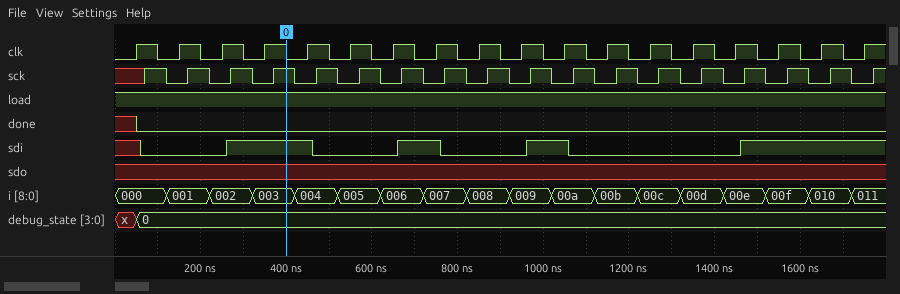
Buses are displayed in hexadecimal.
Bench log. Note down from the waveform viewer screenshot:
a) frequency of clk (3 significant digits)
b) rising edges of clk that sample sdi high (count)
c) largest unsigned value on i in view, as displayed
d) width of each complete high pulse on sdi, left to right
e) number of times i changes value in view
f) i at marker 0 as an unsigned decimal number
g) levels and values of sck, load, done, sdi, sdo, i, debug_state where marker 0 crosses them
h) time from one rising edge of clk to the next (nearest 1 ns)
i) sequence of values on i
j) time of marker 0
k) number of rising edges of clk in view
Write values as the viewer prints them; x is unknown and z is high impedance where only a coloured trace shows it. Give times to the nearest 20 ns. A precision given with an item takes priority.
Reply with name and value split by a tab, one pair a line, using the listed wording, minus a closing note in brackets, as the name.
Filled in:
frequency of clk	10.0 MHz
rising edges of clk that sample sdi high	7
largest unsigned value on i in view, as displayed	011
width of each complete high pulse on sdi, left to right	200 ns, 100 ns, 100 ns
number of times i changes value in view	17
i at marker 0 as an unsigned decimal number	3
levels and values of sck, load, done, sdi, sdo, i, debug_state where marker 0 crosses them	sck=1, load=1, done=0, sdi=1, sdo=x, i=003, debug_state=0
time from one rising edge of clk to the next	100 ns
sequence of values on i	000, 001, 002, 003, 004, 005, 006, 007, 008, 009, 00a, 00b, 00c, 00d, 00e, 00f, 010, 011
time of marker 0	400 ns
number of rising edges of clk in view	18
